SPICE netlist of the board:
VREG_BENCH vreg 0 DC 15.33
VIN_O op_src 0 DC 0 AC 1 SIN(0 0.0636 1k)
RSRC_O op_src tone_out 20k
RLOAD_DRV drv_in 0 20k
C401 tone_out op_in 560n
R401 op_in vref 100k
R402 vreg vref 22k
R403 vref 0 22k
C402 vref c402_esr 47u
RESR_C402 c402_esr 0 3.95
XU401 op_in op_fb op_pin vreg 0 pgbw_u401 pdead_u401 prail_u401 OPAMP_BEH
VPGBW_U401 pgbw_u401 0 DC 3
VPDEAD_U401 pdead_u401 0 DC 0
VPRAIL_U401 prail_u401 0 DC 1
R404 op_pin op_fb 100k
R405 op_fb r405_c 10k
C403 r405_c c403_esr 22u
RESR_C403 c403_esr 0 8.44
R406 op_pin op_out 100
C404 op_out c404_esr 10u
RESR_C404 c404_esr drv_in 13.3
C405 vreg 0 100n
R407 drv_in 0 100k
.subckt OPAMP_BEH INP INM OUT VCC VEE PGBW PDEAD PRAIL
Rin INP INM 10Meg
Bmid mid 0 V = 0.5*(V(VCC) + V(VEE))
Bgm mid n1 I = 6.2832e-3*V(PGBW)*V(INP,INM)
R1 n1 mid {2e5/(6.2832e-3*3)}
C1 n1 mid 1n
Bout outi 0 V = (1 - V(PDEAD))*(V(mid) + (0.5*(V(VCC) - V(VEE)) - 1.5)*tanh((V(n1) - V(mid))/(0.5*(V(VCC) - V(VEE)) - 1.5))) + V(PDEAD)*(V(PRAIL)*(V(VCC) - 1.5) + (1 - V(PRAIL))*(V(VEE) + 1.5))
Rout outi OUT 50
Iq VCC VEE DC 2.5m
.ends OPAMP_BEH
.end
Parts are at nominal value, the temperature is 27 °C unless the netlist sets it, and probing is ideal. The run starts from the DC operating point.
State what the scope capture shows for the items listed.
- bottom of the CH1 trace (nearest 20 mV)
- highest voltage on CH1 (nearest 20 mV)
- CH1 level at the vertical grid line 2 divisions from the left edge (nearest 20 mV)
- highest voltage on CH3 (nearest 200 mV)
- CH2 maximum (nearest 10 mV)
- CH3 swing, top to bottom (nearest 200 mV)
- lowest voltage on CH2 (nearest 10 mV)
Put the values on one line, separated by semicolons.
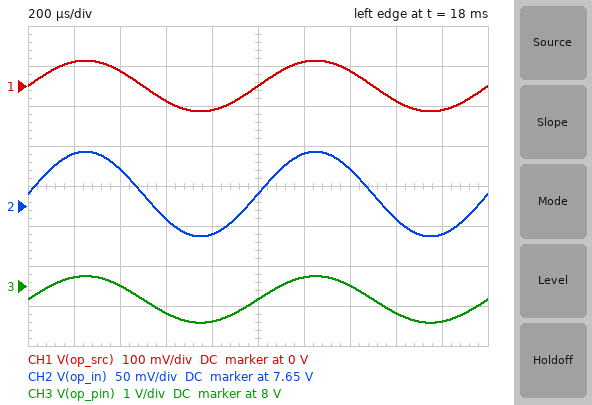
-60 mV; 60 mV; 40 mV; 8.2 V; 7.72 V; 1.2 V; 7.61 V
